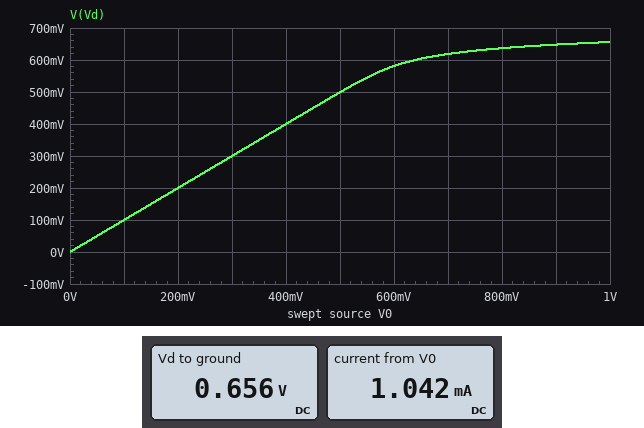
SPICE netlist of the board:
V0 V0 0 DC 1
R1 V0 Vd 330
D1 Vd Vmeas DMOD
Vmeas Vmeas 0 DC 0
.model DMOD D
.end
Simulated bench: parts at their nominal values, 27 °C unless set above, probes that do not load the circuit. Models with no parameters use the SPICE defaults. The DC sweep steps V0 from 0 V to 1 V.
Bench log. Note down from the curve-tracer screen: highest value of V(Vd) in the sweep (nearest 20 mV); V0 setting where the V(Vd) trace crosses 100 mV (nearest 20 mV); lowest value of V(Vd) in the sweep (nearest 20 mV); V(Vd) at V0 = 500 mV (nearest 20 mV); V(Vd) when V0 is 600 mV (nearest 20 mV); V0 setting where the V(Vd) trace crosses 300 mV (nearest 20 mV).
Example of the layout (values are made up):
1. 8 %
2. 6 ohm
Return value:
1. 660 mV
2. 100 mV
3. 0 V
4. 500 mV
5. 580 mV
6. 300 mV
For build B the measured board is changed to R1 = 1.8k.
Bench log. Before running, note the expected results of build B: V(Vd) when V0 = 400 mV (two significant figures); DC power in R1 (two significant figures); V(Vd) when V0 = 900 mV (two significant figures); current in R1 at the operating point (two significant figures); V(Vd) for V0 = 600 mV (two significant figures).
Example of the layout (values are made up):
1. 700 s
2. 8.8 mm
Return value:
1. 400 mV
2. 82 µW
3. 610 mV
4. 210 µA
5. 560 mV
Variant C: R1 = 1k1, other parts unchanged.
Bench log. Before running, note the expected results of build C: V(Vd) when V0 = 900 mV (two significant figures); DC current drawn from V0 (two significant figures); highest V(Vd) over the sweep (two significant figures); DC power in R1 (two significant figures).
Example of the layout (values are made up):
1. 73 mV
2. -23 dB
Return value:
1. 620 mV
2. 340 µA
3. 630 mV
4. 130 µW
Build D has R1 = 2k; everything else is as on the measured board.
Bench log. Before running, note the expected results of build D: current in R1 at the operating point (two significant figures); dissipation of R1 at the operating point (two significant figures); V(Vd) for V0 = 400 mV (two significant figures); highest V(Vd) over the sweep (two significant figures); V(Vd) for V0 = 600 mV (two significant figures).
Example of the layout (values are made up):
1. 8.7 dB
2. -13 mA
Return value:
1. 190 µA
2. 75 µW
3. 400 mV
4. 610 mV
5. 560 mV
